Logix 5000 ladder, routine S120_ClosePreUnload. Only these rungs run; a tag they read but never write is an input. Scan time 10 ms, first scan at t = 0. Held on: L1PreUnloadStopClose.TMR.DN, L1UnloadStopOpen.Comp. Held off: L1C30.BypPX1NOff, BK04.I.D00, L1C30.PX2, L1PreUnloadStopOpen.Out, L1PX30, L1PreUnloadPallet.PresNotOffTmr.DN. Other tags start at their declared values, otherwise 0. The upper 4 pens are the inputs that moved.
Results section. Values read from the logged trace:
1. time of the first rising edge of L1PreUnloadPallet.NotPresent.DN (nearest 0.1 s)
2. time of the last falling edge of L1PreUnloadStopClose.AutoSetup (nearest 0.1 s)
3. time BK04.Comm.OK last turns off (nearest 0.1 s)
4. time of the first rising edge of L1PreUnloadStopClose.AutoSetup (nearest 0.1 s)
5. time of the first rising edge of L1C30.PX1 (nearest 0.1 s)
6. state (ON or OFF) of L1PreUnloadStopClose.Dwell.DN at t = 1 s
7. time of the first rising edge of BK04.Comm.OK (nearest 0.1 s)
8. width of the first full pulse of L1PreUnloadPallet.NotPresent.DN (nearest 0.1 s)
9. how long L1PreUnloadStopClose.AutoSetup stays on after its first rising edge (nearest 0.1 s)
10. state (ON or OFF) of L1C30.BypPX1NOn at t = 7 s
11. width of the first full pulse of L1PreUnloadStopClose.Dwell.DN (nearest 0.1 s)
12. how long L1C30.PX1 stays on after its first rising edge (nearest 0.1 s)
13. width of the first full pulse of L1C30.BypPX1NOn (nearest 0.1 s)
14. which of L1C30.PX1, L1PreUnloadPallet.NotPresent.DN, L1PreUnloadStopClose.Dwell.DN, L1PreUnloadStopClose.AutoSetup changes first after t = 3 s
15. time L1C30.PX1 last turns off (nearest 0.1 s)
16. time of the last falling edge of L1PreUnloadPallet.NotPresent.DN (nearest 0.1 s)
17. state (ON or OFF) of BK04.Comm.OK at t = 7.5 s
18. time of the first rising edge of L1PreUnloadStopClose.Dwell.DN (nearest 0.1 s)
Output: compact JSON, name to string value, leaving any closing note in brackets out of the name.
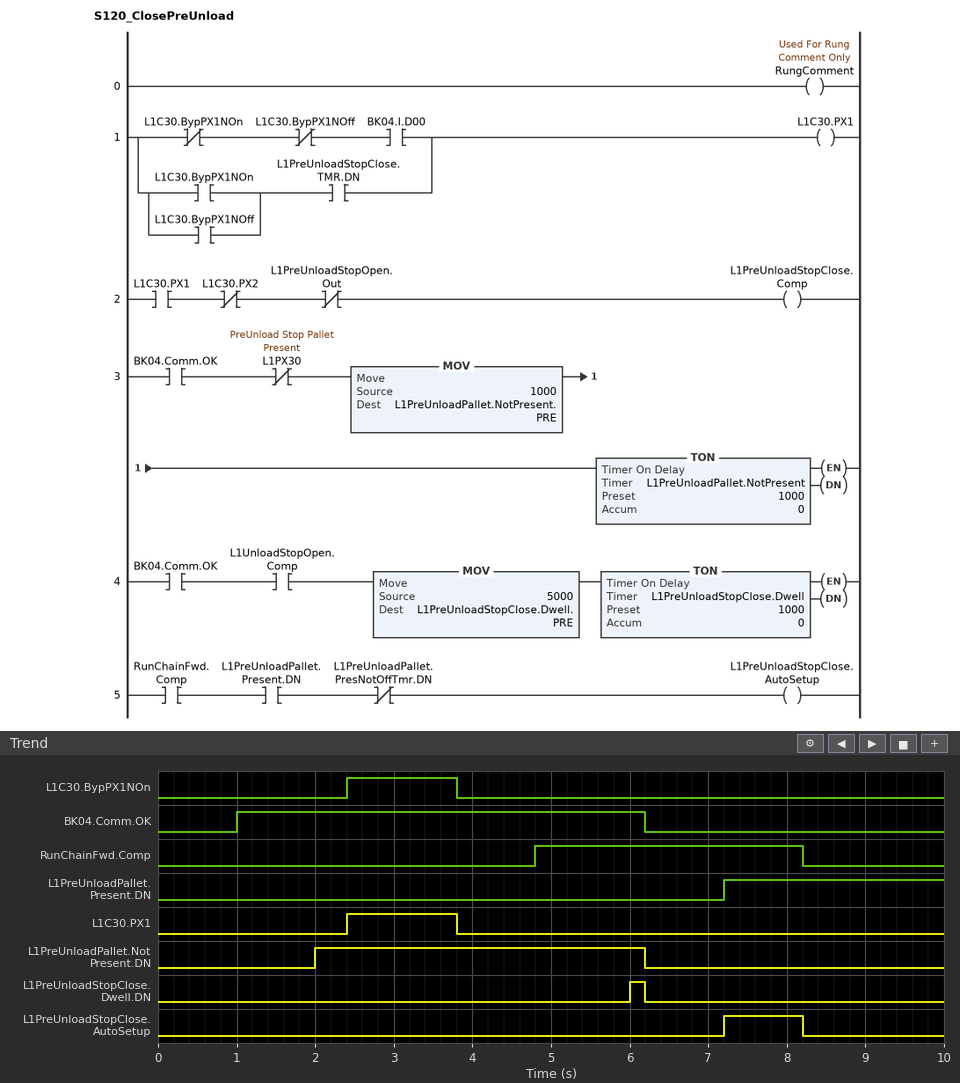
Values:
{"time of the first rising edge of L1PreUnloadPallet.NotPresent.DN": "2.0 s", "time of the last falling edge of L1PreUnloadStopClose.AutoSetup": "8.2 s", "time BK04.Comm.OK last turns off": "6.2 s", "time of the first rising edge of L1PreUnloadStopClose.AutoSetup": "7.2 s", "time of the first rising edge of L1C30.PX1": "2.4 s", "state (ON or OFF) of L1PreUnloadStopClose.Dwell.DN at t = 1 s": "OFF", "time of the first rising edge of BK04.Comm.OK": "1.0 s", "width of the first full pulse of L1PreUnloadPallet.NotPresent.DN": "4.2 s", "how long L1PreUnloadStopClose.AutoSetup stays on after its first rising edge": "1.0 s", "state (ON or OFF) of L1C30.BypPX1NOn at t = 7 s": "OFF", "width of the first full pulse of L1PreUnloadStopClose.Dwell.DN": "0.2 s", "how long L1C30.PX1 stays on after its first rising edge": "1.4 s", "width of the first full pulse of L1C30.BypPX1NOn": "1.4 s", "which of L1C30.PX1, L1PreUnloadPallet.NotPresent.DN, L1PreUnloadStopClose.Dwell.DN, L1PreUnloadStopClose.AutoSetup changes first after t = 3 s": "L1C30.PX1", "time L1C30.PX1 last turns off": "3.8 s", "time of the last falling edge of L1PreUnloadPallet.NotPresent.DN": "6.2 s", "state (ON or OFF) of BK04.Comm.OK at t = 7.5 s": "OFF", "time of the first rising edge of L1PreUnloadStopClose.Dwell.DN": "6.0 s"}
